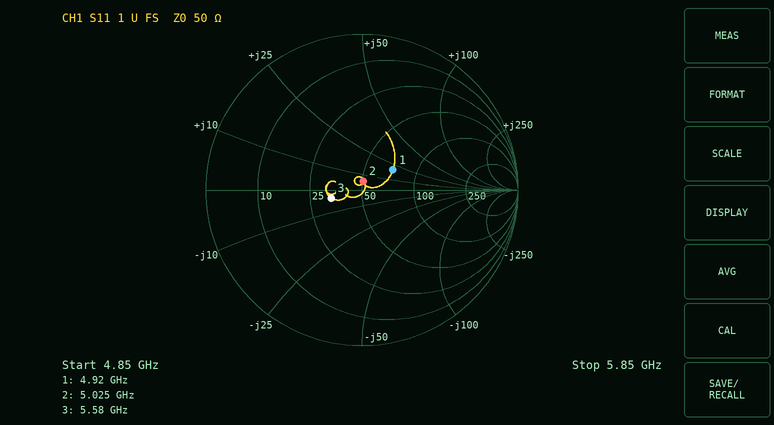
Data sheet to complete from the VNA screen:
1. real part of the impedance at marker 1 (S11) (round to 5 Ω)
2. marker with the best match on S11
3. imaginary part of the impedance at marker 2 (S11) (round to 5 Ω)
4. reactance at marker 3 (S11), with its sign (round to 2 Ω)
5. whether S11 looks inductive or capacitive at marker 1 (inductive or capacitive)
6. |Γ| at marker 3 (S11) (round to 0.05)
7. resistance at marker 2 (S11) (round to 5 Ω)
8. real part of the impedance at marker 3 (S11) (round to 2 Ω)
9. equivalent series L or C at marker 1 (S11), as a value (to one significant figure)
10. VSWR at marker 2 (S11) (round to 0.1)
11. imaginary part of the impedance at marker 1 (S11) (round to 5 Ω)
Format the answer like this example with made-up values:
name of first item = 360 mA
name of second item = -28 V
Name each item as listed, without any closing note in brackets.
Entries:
real part of the impedance at marker 1 (S11) = 70 Ω
marker with the best match on S11 = marker 2
imaginary part of the impedance at marker 2 (S11) = +5 Ω
reactance at marker 3 (S11), with its sign = -4 Ω
whether S11 looks inductive or capacitive at marker 1 = inductive
|Γ| at marker 3 (S11) = 0.20
resistance at marker 2 (S11) = 50 Ω
real part of the impedance at marker 3 (S11) = 34 Ω
equivalent series L or C at marker 1 (S11), as a value = 600 pH
VSWR at marker 2 (S11) = 1.1
imaginary part of the impedance at marker 1 (S11) = +20 Ω
